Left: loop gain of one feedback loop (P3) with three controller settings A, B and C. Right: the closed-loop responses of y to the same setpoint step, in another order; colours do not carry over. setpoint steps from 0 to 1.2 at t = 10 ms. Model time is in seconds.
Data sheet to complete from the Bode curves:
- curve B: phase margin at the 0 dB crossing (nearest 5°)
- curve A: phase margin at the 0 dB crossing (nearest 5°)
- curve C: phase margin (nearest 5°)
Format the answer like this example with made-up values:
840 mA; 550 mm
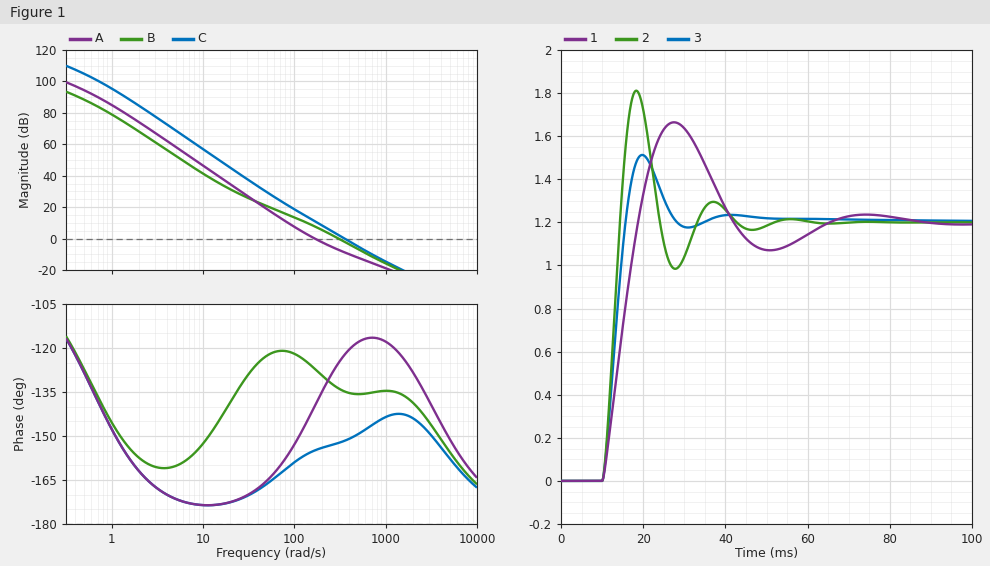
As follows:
45°; 40°; 30°
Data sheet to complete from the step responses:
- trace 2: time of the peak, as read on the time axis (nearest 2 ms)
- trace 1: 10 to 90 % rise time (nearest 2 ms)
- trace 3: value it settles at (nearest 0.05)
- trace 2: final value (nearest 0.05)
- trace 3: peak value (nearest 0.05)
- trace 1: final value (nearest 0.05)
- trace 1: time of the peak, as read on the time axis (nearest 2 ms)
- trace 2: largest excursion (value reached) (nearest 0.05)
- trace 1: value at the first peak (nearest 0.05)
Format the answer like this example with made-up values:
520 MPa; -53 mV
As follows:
18 ms; 6 ms; 1.20; 1.20; 1.50; 1.20; 28 ms; 1.80; 1.65
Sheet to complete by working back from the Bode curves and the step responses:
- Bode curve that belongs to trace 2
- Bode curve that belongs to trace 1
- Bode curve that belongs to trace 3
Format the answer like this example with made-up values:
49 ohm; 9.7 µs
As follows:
C; A; B
